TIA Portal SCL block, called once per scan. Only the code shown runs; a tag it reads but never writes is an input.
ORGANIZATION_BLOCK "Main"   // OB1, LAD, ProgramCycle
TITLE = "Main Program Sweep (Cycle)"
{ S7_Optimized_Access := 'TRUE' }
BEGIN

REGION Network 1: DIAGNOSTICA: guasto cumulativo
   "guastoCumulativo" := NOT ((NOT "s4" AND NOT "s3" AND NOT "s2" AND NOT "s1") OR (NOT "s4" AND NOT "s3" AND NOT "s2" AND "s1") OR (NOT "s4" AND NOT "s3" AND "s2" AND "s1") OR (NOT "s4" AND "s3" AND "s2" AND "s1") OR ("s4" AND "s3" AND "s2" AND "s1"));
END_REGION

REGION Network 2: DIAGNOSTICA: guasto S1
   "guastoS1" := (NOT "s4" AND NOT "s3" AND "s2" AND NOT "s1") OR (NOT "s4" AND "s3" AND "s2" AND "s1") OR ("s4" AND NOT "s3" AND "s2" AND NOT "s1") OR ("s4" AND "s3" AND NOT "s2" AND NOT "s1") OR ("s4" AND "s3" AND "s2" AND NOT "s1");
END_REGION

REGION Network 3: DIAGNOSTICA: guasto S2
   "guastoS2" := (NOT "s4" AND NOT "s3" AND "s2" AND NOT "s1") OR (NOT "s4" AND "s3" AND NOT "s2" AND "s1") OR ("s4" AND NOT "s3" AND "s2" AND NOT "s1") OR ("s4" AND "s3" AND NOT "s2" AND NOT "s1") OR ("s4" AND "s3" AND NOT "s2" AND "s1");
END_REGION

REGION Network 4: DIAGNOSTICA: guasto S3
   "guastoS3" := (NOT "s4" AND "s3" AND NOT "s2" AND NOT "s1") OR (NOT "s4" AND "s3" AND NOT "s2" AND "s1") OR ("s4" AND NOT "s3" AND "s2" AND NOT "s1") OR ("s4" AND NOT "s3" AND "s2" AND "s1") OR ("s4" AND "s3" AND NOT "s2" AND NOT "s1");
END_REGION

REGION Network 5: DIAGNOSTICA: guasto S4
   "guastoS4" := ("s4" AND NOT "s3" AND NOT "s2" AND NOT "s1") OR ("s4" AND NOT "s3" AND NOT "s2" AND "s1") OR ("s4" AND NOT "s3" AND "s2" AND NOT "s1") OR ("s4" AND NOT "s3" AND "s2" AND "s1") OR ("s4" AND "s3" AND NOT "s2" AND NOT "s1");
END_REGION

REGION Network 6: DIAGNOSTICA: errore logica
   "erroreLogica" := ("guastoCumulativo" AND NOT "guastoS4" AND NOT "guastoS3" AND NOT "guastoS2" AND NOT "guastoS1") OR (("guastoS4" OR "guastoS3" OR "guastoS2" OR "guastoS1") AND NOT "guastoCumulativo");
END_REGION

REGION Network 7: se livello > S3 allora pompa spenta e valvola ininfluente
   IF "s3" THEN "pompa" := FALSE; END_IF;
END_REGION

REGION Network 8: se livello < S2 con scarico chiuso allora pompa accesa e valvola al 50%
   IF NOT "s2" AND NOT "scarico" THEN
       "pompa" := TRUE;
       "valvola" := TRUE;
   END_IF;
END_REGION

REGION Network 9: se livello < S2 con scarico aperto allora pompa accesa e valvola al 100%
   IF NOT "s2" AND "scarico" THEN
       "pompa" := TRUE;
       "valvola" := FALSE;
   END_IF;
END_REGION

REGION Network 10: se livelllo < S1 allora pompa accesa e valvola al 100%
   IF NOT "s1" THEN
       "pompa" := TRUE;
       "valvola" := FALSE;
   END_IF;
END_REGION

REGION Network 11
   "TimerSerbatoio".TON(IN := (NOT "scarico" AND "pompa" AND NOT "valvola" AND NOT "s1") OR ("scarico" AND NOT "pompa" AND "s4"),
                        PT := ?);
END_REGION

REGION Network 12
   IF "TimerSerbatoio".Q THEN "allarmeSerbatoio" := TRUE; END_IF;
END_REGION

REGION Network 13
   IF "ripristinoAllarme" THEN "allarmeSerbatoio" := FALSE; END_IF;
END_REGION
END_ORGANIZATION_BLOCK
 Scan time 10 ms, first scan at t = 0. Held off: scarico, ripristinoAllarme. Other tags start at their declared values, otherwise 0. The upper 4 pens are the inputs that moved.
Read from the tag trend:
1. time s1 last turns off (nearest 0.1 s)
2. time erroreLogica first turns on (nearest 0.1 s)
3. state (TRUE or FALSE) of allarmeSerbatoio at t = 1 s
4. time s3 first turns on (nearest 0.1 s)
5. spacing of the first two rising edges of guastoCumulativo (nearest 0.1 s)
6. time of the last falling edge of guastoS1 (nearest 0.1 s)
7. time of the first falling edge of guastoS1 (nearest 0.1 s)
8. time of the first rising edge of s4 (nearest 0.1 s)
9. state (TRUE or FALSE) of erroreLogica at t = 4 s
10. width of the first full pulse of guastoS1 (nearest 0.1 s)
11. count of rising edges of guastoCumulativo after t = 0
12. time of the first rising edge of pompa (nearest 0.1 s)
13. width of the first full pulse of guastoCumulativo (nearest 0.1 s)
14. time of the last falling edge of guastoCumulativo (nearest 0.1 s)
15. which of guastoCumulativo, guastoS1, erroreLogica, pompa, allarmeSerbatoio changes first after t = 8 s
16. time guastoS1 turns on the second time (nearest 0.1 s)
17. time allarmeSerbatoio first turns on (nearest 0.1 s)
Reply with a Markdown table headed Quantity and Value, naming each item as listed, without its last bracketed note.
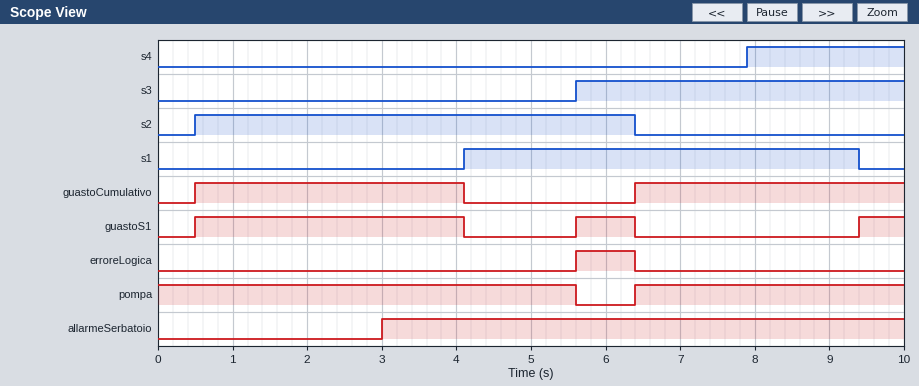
| Quantity | Value |
|---|---|
| time s1 last turns off | 9.4 s |
| time erroreLogica first turns on | 5.6 s |
| state (TRUE or FALSE) of allarmeSerbatoio at t = 1 s | FALSE |
| time s3 first turns on | 5.6 s |
| spacing of the first two rising edges of guastoCumulativo | 5.9 s |
| time of the last falling edge of guastoS1 | 6.4 s |
| time of the first falling edge of guastoS1 | 4.1 s |
| time of the first rising edge of s4 | 7.9 s |
| state (TRUE or FALSE) of erroreLogica at t = 4 s | FALSE |
| width of the first full pulse of guastoS1 | 3.6 s |
| count of rising edges of guastoCumulativo after t = 0 | 2 |
| time of the first rising edge of pompa | 6.4 s |
| width of the first full pulse of guastoCumulativo | 3.6 s |
| time of the last falling edge of guastoCumulativo | 4.1 s |
| which of guastoCumulativo, guastoS1, erroreLogica, pompa, allarmeSerbatoio changes first after t = 8 s | guastoS1 |
| time guastoS1 turns on the second time | 5.6 s |
| time allarmeSerbatoio first turns on | 3.0 s |
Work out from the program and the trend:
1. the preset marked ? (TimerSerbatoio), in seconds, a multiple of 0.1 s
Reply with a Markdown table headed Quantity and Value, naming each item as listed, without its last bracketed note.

| Quantity | Value |
|---|---|
| the preset marked ? (TimerSerbatoio), in seconds, a multiple of 0.1 s | 3.0 s |
